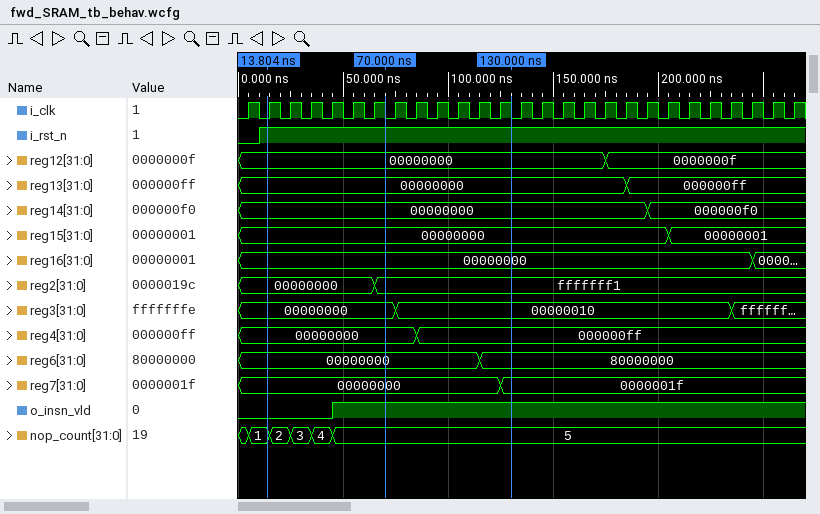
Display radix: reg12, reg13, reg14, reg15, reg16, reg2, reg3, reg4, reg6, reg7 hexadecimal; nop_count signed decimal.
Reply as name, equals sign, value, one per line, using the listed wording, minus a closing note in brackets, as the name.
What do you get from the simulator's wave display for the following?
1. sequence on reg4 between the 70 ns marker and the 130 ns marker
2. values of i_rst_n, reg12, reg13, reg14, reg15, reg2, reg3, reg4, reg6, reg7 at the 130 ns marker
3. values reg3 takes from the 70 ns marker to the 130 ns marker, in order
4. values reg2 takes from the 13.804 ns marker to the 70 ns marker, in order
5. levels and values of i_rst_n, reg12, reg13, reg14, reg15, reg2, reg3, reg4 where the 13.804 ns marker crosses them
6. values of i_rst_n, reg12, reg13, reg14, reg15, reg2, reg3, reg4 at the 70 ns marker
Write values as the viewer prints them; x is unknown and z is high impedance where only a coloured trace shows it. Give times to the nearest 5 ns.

sequence on reg4 between the 70 ns marker and the 130 ns marker = 00000000, 000000ff
values of i_rst_n, reg12, reg13, reg14, reg15, reg2, reg3, reg4, reg6, reg7 at the 130 ns marker = i_rst_n=1, reg12=00000000, reg13=00000000, reg14=00000000, reg15=00000000, reg2=fffffff1, reg3=00000010, reg4=000000ff, reg6=80000000, reg7=0000001f
values reg3 takes from the 70 ns marker to the 130 ns marker, in order = 00000000, 00000010
values reg2 takes from the 13.804 ns marker to the 70 ns marker, in order = 00000000, fffffff1
levels and values of i_rst_n, reg12, reg13, reg14, reg15, reg2, reg3, reg4 where the 13.804 ns marker crosses them = i_rst_n=1, reg12=00000000, reg13=00000000, reg14=00000000, reg15=00000000, reg2=00000000, reg3=00000000, reg4=00000000
values of i_rst_n, reg12, reg13, reg14, reg15, reg2, reg3, reg4 at the 70 ns marker = i_rst_n=1, reg12=00000000, reg13=00000000, reg14=00000000, reg15=00000000, reg2=fffffff1, reg3=00000000, reg4=00000000
